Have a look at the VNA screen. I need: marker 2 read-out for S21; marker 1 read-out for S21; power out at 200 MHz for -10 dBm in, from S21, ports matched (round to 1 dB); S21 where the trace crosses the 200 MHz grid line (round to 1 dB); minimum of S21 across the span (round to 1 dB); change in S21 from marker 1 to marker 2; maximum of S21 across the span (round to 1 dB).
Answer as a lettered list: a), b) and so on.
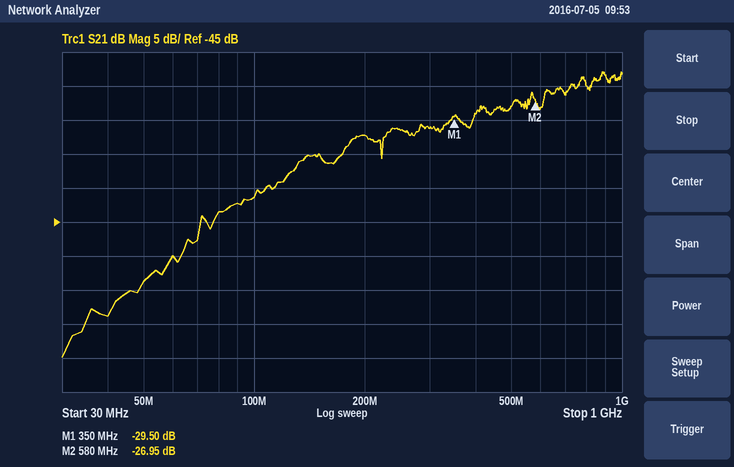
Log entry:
a) -26.95 dB
b) -29.50 dB
c) -42 dBm
d) -32 dB
e) -65 dB
f) 2.55 dB
g) -23 dB
